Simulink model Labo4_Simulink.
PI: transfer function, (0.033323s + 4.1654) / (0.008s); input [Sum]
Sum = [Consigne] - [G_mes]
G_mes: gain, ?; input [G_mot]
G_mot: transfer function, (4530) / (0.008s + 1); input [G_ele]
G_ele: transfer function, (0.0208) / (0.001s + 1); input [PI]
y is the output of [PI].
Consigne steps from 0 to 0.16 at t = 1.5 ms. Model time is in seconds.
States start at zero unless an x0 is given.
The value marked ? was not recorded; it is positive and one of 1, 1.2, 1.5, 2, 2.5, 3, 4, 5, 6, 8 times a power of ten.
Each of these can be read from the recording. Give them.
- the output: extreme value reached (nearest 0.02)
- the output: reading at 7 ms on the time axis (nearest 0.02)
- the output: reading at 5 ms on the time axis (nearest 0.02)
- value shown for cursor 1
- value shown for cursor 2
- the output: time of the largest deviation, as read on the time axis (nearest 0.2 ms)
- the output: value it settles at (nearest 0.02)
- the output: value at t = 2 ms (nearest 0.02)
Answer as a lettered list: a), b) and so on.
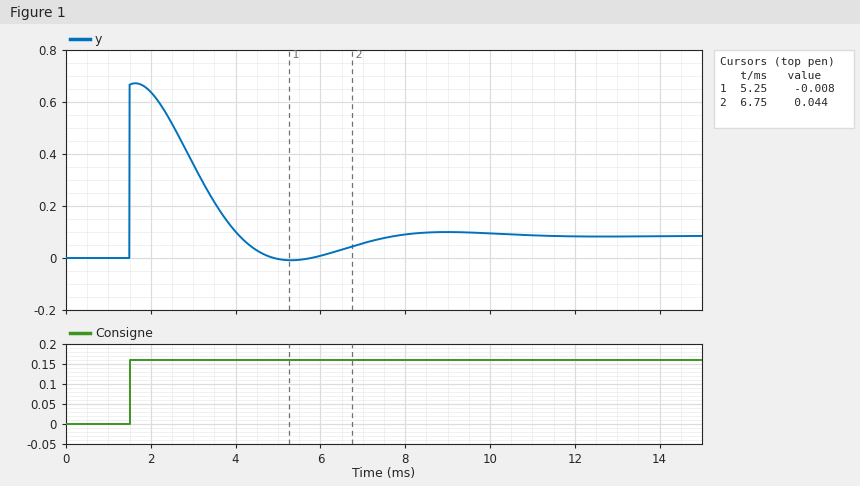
a) 0.68
b) 0.06
c) 0.00
d) -0.008
e) 0.044
f) 1.6 ms
g) 0.08
h) 0.64
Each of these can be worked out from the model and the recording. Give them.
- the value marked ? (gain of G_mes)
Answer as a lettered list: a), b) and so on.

a) 0.02
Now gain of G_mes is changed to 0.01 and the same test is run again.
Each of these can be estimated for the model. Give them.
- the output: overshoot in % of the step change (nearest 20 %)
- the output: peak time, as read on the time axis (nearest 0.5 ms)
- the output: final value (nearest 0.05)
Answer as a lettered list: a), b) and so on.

a) 300 %
b) 2.0 ms
c) 0.15
